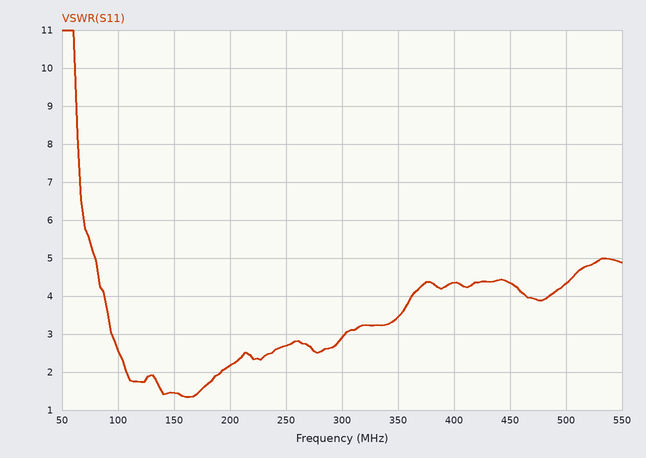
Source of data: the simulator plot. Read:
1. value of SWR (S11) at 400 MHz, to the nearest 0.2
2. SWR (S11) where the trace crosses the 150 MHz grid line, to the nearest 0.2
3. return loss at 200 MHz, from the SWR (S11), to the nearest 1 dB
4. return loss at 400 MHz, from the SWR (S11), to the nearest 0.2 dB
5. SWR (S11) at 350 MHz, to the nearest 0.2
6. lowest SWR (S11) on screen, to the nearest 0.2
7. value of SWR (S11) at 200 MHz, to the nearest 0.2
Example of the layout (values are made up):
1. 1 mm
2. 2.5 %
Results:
1. 4.4
2. 1.4
3. 9 dB
4. 4.0 dB
5. 3.4
6. 1.4
7. 2.2
